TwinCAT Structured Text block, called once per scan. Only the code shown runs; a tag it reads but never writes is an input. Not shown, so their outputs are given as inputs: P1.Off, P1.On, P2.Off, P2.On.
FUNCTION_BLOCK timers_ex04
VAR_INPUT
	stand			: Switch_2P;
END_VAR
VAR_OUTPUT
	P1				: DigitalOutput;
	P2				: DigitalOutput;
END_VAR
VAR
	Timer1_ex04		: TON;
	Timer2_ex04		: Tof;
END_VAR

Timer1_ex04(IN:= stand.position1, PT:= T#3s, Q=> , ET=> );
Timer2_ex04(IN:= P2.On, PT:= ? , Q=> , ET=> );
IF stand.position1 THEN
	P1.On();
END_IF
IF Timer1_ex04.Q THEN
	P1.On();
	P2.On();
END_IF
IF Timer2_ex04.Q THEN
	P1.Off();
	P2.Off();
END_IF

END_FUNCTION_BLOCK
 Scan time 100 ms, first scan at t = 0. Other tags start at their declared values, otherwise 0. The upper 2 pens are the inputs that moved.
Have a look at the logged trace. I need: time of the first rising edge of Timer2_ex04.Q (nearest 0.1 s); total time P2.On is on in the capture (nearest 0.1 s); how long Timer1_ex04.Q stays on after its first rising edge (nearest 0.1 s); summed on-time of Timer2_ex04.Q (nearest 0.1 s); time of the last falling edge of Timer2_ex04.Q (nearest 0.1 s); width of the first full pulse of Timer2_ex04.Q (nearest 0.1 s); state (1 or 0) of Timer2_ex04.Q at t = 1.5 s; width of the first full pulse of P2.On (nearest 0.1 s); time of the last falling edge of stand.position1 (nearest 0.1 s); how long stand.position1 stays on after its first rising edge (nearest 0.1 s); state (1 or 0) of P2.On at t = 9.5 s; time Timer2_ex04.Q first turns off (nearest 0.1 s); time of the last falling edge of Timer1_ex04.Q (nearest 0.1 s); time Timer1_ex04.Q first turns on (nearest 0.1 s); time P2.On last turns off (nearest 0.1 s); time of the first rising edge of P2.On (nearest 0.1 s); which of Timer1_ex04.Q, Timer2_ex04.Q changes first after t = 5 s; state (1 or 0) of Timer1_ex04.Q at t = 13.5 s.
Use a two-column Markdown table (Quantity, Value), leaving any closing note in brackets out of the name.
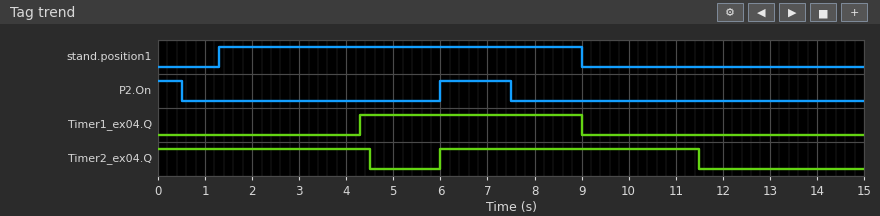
| Quantity | Value |
|---|---|
| time of the first rising edge of Timer2_ex04.Q | 6.0 s |
| total time P2.On is on in the capture | 2.0 s |
| how long Timer1_ex04.Q stays on after its first rising edge | 4.7 s |
| summed on-time of Timer2_ex04.Q | 10.0 s |
| time of the last falling edge of Timer2_ex04.Q | 11.5 s |
| width of the first full pulse of Timer2_ex04.Q | 5.5 s |
| state (1 or 0) of Timer2_ex04.Q at t = 1.5 s | 1 |
| width of the first full pulse of P2.On | 1.5 s |
| time of the last falling edge of stand.position1 | 9.0 s |
| how long stand.position1 stays on after its first rising edge | 7.7 s |
| state (1 or 0) of P2.On at t = 9.5 s | 0 |
| time Timer2_ex04.Q first turns off | 4.5 s |
| time of the last falling edge of Timer1_ex04.Q | 9.0 s |
| time Timer1_ex04.Q first turns on | 4.3 s |
| time P2.On last turns off | 7.5 s |
| time of the first rising edge of P2.On | 6.0 s |
| which of Timer1_ex04.Q, Timer2_ex04.Q changes first after t = 5 s | Timer2_ex04.Q |
| state (1 or 0) of Timer1_ex04.Q at t = 13.5 s | 0 |
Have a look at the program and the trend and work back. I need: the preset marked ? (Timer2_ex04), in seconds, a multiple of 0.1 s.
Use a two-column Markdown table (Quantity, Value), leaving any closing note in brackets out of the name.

| Quantity | Value |
|---|---|
| the preset marked ? (Timer2_ex04), in seconds, a multiple of 0.1 s | 4.0 s |
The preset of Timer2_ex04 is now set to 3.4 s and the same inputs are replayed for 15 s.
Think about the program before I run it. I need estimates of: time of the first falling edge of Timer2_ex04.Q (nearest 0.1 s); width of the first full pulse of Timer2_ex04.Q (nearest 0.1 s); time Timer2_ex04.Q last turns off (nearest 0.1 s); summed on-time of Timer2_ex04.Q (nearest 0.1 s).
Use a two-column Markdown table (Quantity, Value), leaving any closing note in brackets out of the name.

| Quantity | Value |
|---|---|
| time of the first falling edge of Timer2_ex04.Q | 3.9 s |
| width of the first full pulse of Timer2_ex04.Q | 4.9 s |
| time Timer2_ex04.Q last turns off | 10.9 s |
| summed on-time of Timer2_ex04.Q | 8.8 s |
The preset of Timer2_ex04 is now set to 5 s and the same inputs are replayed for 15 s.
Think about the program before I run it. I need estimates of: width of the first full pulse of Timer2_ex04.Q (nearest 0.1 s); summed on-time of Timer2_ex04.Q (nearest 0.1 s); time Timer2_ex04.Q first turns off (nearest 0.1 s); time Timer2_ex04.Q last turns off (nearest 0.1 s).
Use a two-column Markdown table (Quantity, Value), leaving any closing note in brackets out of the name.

| Quantity | Value |
|---|---|
| width of the first full pulse of Timer2_ex04.Q | 6.5 s |
| summed on-time of Timer2_ex04.Q | 12.0 s |
| time Timer2_ex04.Q first turns off | 5.5 s |
| time Timer2_ex04.Q last turns off | 12.5 s |
